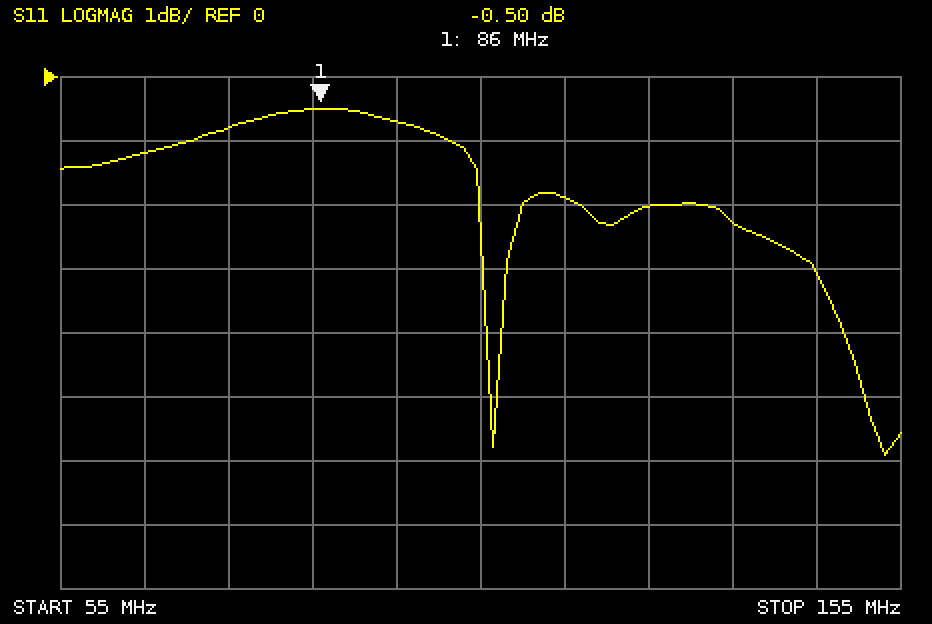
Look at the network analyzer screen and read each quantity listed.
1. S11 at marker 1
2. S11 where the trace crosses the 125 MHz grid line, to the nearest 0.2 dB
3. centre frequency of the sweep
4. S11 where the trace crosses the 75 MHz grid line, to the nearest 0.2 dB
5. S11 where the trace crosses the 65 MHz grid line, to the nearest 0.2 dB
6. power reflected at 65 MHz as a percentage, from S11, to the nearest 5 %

-0.50 dB
-2.0 dB
105 MHz
-0.8 dB
-1.2 dB
75 %
